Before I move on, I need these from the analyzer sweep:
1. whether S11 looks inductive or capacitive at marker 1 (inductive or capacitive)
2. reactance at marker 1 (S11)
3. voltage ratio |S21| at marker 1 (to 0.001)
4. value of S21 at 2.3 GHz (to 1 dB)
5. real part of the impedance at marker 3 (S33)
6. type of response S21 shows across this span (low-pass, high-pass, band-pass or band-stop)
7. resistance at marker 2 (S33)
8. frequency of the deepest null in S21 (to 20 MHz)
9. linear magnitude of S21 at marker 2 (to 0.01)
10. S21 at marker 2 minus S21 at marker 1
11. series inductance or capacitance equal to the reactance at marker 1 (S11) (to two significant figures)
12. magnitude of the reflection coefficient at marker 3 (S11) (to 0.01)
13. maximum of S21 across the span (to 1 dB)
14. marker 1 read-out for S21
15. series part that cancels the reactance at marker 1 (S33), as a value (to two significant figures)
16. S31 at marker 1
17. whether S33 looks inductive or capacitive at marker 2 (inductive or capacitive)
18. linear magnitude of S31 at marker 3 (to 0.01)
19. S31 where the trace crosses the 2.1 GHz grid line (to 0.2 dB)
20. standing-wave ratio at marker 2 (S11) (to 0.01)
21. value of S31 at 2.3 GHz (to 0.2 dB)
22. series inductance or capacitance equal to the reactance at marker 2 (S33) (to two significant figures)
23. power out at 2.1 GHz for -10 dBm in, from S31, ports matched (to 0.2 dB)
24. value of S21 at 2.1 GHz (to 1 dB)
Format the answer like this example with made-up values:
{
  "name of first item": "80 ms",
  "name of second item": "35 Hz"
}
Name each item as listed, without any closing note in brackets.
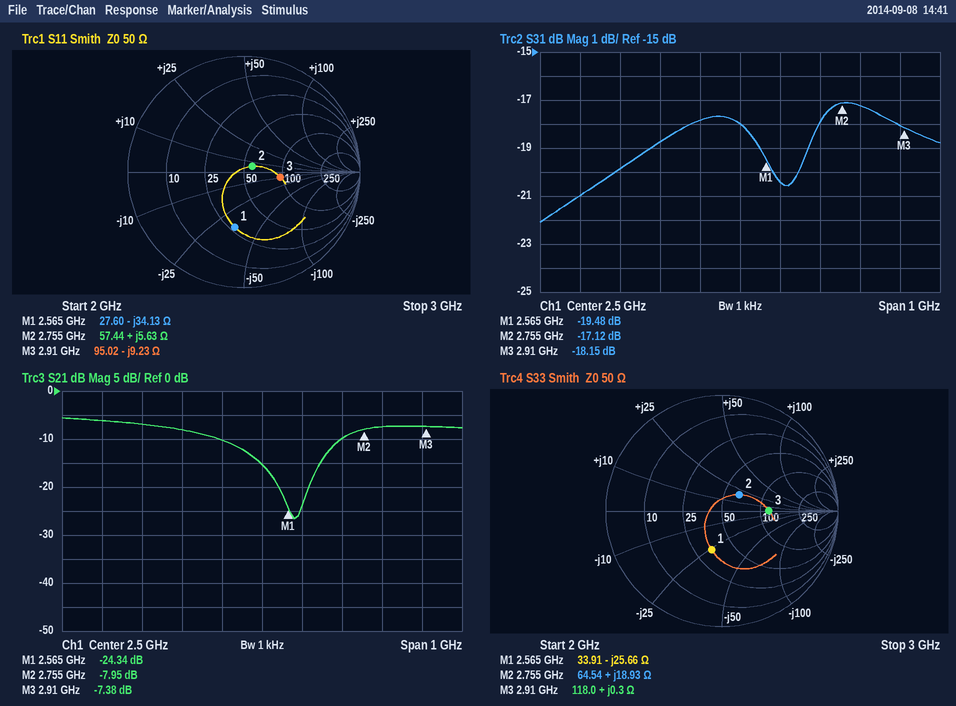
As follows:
{
  "whether S11 looks inductive or capacitive at marker 1": "capacitive",
  "reactance at marker 1": "-34.13 Ω",
  "voltage ratio |S21| at marker 1": "0.061",
  "value of S21 at 2.3 GHz": "-8 dB",
  "real part of the impedance at marker 3": "118.0 Ω",
  "type of response S21 shows across this span": "band-stop",
  "resistance at marker 2": "64.54 Ω",
  "frequency of the deepest null in S21": "2.58 GHz",
  "linear magnitude of S21 at marker 2": "0.40",
  "S21 at marker 2 minus S21 at marker 1": "16.39 dB",
  "series inductance or capacitance equal to the reactance at marker 1 (S11)": "1.8 pF",
  "magnitude of the reflection coefficient at marker 3 (S11)": "0.32",
  "maximum of S21 across the span": "-6 dB",
  "marker 1 read-out for S21": "-24.34 dB",
  "series part that cancels the reactance at marker 1 (S33), as a value": "1.6 nH",
  "S31 at marker 1": "-19.48 dB",
  "whether S33 looks inductive or capacitive at marker 2": "inductive",
  "linear magnitude of S31 at marker 3": "0.12",
  "S31 where the trace crosses the 2.1 GHz grid line": "-21.0 dB",
  "standing-wave ratio at marker 2 (S11)": "1.19",
  "value of S31 at 2.3 GHz": "-18.8 dB",
  "series inductance or capacitance equal to the reactance at marker 2 (S33)": "1.1 nH",
  "power out at 2.1 GHz for -10 dBm in, from S31, ports matched": "-31.0 dBm",
  "value of S21 at 2.1 GHz": "-6 dB"
}
